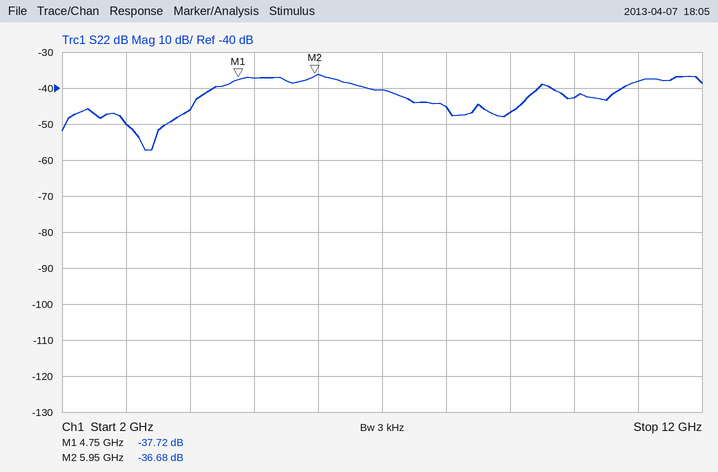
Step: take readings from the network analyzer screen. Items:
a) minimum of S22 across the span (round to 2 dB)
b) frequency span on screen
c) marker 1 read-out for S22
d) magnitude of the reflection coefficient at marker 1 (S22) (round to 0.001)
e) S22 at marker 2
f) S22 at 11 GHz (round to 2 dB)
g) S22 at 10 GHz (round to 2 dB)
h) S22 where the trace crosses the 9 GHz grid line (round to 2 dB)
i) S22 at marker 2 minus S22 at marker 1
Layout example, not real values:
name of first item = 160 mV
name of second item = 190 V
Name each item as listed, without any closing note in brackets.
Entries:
minimum of S22 across the span = -58 dB
frequency span on screen = 10 GHz
marker 1 read-out for S22 = -37.72 dB
magnitude of the reflection coefficient at marker 1 (S22) = 0.013
S22 at marker 2 = -36.68 dB
S22 at 11 GHz = -38 dB
S22 at 10 GHz = -42 dB
S22 where the trace crosses the 9 GHz grid line = -46 dB
S22 at marker 2 minus S22 at marker 1 = 1.04 dB
